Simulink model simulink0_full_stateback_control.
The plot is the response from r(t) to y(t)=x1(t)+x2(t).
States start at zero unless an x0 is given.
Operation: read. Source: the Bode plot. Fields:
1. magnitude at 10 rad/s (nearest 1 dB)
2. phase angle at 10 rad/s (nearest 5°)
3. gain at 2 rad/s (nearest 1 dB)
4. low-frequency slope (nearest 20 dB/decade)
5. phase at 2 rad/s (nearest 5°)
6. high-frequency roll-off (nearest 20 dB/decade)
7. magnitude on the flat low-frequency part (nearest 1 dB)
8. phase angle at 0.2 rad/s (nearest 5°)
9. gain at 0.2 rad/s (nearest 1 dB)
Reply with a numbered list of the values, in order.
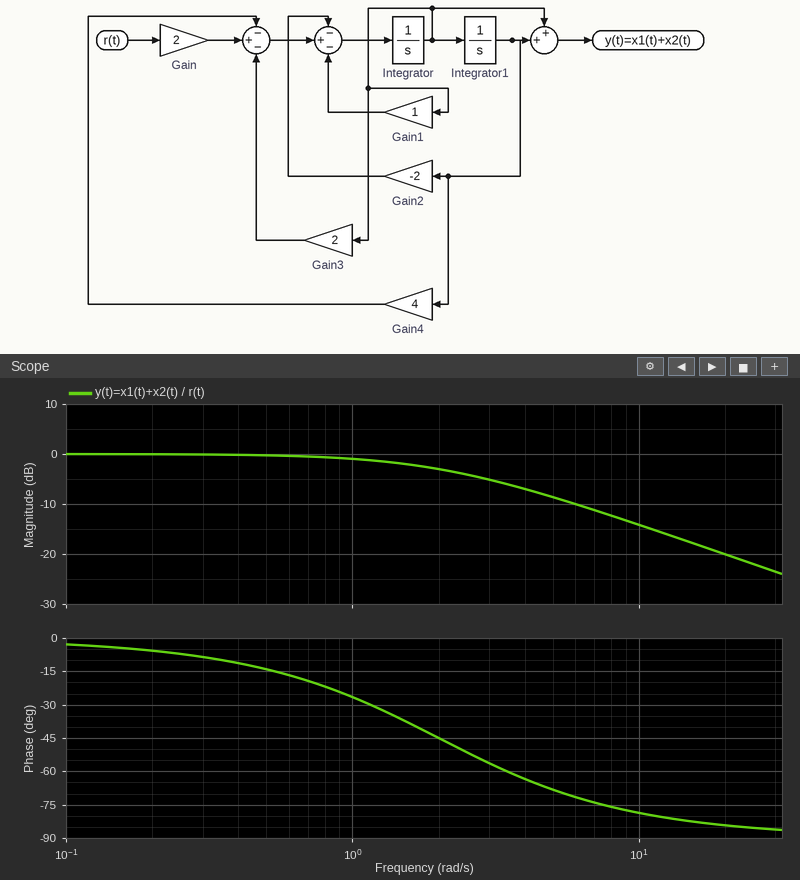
1. -14 dB
2. -80°
3. -3 dB
4. 0 dB/decade
5. -45°
6. -20 dB/decade
7. 0 dB
8. -5°
9. 0 dB
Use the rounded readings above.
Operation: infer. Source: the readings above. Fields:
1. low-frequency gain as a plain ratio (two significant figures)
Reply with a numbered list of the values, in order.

1. 1.0
